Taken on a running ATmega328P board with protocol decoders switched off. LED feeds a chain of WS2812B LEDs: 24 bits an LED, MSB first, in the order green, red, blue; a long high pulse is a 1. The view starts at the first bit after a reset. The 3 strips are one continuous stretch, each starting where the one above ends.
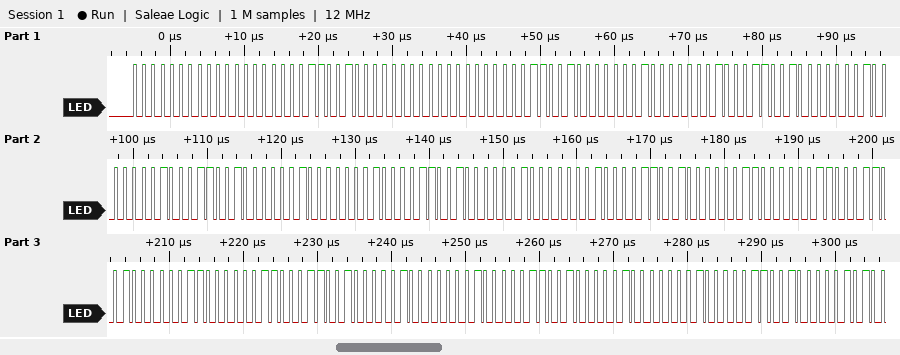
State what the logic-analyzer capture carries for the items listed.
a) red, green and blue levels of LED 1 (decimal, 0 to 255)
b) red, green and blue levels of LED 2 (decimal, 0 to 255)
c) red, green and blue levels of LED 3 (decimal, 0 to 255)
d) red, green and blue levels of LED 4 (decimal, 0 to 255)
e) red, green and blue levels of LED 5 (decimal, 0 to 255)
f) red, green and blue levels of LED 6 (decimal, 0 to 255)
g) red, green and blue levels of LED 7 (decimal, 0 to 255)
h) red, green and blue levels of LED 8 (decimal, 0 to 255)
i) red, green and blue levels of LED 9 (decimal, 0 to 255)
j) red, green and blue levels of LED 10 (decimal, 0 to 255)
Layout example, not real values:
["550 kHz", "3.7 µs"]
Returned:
["0, 0, 25", "0, 0, 25", "1, 1, 25", "1, 1, 25", "2, 2, 25", "2, 2, 25", "3, 3, 25", "3, 3, 25", "4, 4, 25", "4, 4, 25"]
